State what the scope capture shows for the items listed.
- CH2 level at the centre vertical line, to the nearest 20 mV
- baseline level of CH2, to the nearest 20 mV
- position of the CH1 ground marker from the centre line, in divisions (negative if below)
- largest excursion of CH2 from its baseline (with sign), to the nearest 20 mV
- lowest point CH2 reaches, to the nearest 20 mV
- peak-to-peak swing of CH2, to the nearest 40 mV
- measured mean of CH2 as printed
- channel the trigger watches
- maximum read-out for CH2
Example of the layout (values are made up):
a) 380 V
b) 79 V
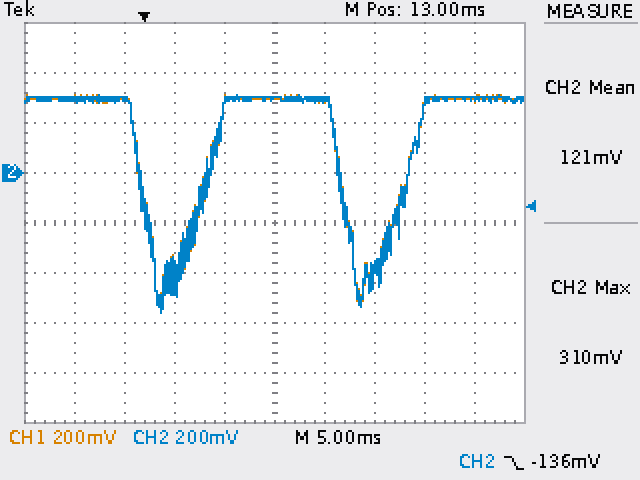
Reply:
a) 300 mV
b) 300 mV
c) +1.0 div
d) -860 mV
e) -560 mV
f) 880 mV
g) 121 mV
h) CH2
i) 310 mV
